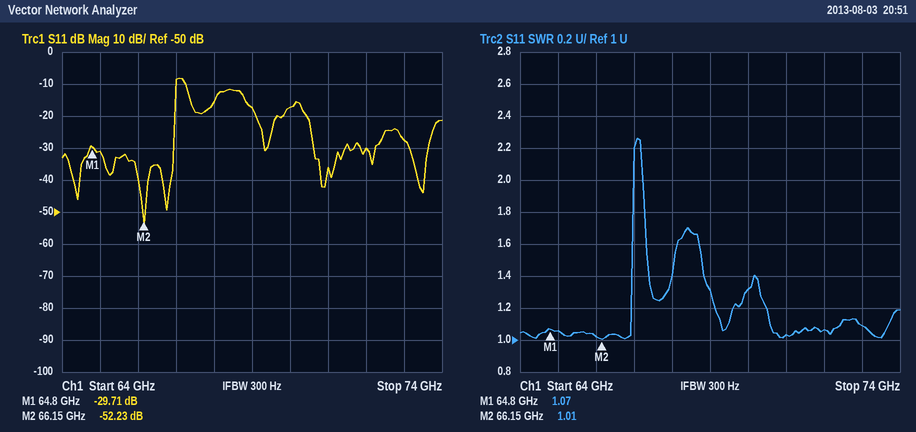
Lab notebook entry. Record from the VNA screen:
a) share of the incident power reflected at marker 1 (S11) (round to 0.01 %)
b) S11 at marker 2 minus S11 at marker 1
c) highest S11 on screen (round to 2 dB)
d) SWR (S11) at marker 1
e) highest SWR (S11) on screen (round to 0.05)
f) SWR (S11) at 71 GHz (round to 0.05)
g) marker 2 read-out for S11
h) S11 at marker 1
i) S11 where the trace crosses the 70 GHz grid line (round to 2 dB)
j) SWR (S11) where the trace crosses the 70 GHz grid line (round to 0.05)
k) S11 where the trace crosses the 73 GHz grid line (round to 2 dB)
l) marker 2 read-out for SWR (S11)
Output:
0.11 %
-22.52 dB
-8 dB
1.07
2.25
1.05
-52.23 dB
-29.71 dB
-18 dB
1.30
-28 dB
1.01
